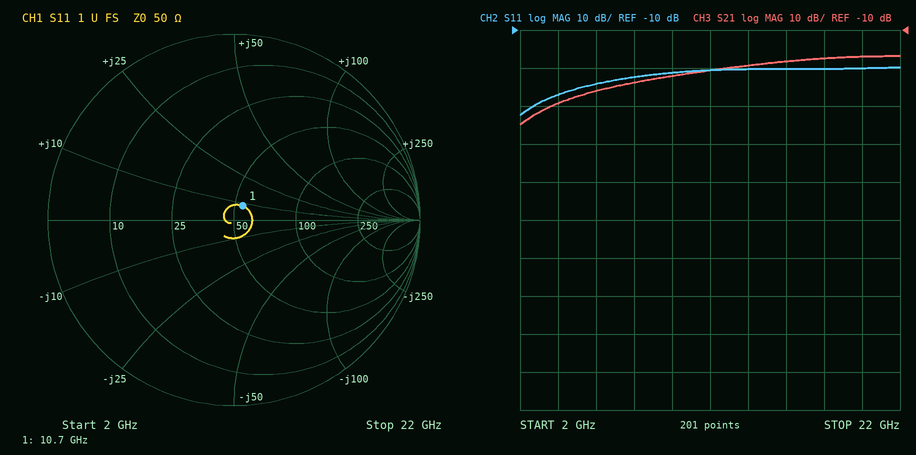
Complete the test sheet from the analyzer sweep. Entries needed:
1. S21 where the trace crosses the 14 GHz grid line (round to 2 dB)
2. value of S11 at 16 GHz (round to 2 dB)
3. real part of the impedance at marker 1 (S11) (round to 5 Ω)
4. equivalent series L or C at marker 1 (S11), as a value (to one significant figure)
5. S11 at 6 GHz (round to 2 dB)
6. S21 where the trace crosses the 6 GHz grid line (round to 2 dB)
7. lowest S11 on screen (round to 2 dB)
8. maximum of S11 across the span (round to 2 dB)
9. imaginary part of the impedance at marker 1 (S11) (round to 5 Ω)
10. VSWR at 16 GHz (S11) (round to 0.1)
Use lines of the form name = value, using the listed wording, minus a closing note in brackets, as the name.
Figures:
S21 where the trace crosses the 14 GHz grid line = -20 dB
value of S11 at 16 GHz = -20 dB
real part of the impedance at marker 1 (S11) = 55 Ω
equivalent series L or C at marker 1 (S11), as a value = 100 pH
S11 at 6 GHz = -24 dB
S21 where the trace crosses the 6 GHz grid line = -26 dB
lowest S11 on screen = -32 dB
maximum of S11 across the span = -20 dB
imaginary part of the impedance at marker 1 (S11) = +10 Ω
VSWR at 16 GHz (S11) = 1.2
